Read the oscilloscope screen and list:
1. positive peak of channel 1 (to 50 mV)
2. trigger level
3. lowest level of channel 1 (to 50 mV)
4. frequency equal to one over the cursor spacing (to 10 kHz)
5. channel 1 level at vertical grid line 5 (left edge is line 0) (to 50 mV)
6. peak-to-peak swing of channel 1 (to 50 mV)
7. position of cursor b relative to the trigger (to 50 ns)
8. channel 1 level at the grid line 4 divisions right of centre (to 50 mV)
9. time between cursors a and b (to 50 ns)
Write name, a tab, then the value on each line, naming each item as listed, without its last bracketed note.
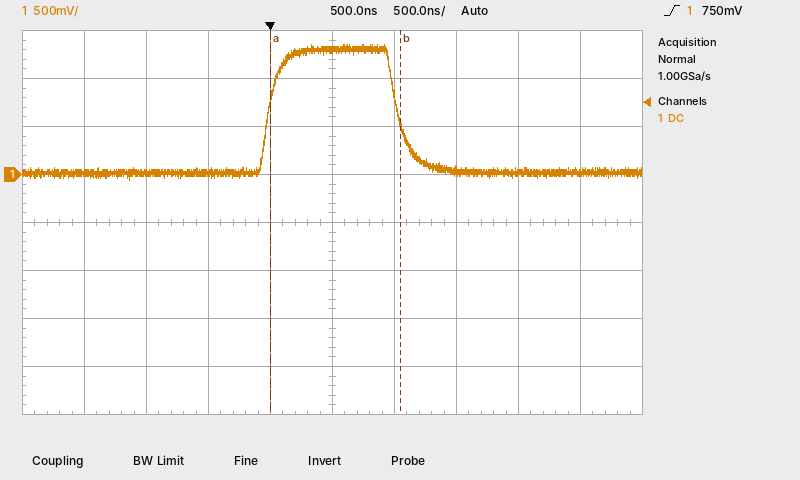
positive peak of channel 1	1.35 V
trigger level	750 mV
lowest level of channel 1	-50 mV
frequency equal to one over the cursor spacing	950 kHz
channel 1 level at vertical grid line 5 (left edge is line 0)	1.30 V
peak-to-peak swing of channel 1	1.40 V
position of cursor b relative to the trigger	+1.05 µs
channel 1 level at the grid line 4 divisions right of centre	50 mV
time between cursors a and b	1.05 µs
